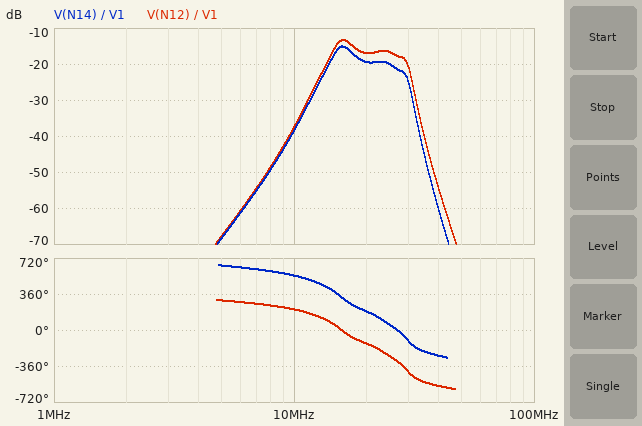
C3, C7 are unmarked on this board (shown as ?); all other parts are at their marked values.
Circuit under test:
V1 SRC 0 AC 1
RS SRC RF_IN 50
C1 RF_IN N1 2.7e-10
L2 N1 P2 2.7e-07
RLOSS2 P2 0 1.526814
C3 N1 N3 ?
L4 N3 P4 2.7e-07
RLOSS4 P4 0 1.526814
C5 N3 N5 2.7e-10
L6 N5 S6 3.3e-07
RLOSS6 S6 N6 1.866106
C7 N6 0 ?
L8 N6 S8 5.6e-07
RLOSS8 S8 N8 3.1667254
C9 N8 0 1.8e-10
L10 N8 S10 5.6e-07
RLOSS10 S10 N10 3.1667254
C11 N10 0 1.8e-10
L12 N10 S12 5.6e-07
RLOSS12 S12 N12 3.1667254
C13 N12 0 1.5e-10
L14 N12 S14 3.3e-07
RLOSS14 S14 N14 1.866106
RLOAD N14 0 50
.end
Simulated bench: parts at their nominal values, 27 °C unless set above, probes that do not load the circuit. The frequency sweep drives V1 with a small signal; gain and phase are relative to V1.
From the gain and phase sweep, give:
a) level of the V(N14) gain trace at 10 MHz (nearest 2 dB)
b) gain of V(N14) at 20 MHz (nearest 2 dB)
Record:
-38 dB
-20 dB
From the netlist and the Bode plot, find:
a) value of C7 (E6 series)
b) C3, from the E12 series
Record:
470 pF
68 pF
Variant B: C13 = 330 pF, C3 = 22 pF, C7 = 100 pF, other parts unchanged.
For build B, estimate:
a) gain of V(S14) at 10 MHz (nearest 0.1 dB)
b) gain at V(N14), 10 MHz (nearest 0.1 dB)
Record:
-47.2 dB
-47.5 dB
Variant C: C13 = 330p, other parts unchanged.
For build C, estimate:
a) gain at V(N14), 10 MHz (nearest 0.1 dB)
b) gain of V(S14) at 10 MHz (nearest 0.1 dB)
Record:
-39.8 dB
-39.5 dB
